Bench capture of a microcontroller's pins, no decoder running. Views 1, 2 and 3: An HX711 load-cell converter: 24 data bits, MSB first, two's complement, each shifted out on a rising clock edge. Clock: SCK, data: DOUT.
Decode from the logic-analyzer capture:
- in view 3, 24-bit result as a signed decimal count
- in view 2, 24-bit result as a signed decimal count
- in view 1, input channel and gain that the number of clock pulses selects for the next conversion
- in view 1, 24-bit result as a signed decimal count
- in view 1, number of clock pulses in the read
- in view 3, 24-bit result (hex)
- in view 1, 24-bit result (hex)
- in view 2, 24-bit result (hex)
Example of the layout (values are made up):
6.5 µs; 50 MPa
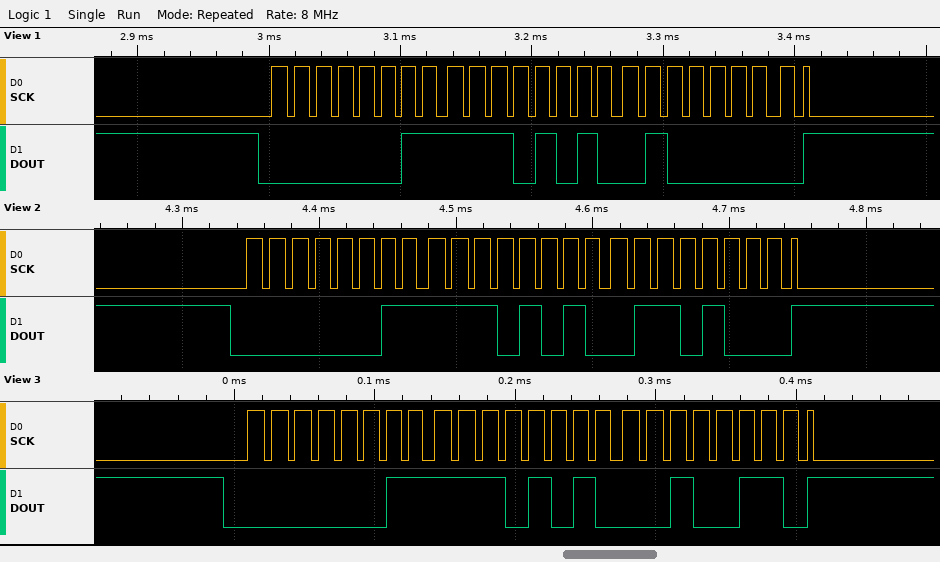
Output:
256550; 256616; channel A, gain 128; 256576; 25; 0x03EA26; 0x03EA40; 0x03EA68
